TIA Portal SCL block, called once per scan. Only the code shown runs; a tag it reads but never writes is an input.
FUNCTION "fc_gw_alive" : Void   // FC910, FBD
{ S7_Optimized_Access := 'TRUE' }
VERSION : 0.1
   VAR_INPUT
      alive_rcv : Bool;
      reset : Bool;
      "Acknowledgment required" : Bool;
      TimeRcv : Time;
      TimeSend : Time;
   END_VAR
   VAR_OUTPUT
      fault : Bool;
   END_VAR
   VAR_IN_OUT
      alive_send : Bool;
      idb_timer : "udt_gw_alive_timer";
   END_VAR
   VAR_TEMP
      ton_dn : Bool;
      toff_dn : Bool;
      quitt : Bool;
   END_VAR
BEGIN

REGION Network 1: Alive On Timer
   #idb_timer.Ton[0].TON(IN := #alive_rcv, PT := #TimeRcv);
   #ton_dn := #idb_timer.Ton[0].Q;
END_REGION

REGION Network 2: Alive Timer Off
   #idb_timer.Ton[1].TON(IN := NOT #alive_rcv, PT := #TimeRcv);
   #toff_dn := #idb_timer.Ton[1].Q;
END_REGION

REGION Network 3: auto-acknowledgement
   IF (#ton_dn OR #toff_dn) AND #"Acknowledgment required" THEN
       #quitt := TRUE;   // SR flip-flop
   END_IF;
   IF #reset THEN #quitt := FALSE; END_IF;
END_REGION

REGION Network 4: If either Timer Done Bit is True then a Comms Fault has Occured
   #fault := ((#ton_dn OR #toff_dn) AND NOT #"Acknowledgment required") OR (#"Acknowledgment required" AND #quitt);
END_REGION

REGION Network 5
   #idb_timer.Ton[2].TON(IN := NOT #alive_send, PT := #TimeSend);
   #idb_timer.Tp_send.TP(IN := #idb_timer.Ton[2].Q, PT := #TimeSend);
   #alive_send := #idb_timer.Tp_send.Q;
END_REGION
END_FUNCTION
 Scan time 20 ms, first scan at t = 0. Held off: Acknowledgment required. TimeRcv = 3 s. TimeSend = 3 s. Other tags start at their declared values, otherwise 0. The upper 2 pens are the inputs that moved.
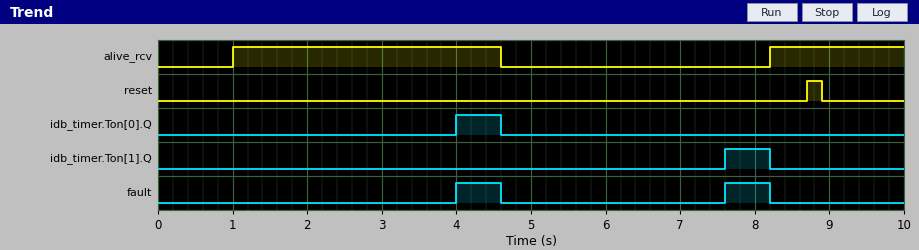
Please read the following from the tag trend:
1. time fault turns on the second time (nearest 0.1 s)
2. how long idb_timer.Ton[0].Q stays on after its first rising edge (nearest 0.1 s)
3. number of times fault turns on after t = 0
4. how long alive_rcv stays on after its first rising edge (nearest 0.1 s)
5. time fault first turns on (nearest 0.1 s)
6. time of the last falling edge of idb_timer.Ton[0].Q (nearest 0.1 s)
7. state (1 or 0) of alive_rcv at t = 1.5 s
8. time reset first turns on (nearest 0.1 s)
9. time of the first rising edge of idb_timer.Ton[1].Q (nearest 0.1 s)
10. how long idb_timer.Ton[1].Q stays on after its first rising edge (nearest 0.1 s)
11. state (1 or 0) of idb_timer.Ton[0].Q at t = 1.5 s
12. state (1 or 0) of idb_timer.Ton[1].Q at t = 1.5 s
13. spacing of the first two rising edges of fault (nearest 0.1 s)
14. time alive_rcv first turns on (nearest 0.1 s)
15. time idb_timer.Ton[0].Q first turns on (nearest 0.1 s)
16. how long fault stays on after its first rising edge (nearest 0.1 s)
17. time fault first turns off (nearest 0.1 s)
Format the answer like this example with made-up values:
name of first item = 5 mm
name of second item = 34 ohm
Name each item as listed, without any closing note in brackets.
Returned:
time fault turns on the second time = 7.6 s
how long idb_timer.Ton[0].Q stays on after its first rising edge = 0.6 s
number of times fault turns on after t = 0 = 2
how long alive_rcv stays on after its first rising edge = 3.6 s
time fault first turns on = 4.0 s
time of the last falling edge of idb_timer.Ton[0].Q = 4.6 s
state (1 or 0) of alive_rcv at t = 1.5 s = 1
time reset first turns on = 8.7 s
time of the first rising edge of idb_timer.Ton[1].Q = 7.6 s
how long idb_timer.Ton[1].Q stays on after its first rising edge = 0.6 s
state (1 or 0) of idb_timer.Ton[0].Q at t = 1.5 s = 0
state (1 or 0) of idb_timer.Ton[1].Q at t = 1.5 s = 0
spacing of the first two rising edges of fault = 3.6 s
time alive_rcv first turns on = 1.0 s
time idb_timer.Ton[0].Q first turns on = 4.0 s
how long fault stays on after its first rising edge = 0.6 s
time fault first turns off = 4.6 s
